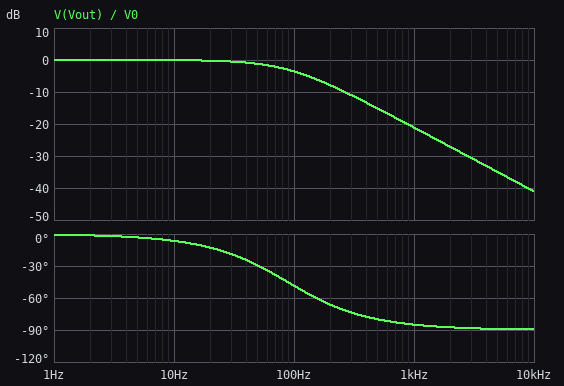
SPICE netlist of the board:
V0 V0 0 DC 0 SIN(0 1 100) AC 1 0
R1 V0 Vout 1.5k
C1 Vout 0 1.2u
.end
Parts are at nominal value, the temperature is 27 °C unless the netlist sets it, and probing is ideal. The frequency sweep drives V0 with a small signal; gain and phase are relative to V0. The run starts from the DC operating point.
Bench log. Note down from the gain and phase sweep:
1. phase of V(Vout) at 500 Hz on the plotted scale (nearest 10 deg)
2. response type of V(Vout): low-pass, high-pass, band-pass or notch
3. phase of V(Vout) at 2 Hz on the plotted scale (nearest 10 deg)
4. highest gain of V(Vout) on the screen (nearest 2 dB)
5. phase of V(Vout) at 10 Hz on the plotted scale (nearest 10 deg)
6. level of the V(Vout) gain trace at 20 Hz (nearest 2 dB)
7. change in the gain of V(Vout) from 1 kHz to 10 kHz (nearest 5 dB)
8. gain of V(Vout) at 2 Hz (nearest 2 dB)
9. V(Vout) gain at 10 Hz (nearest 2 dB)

-80 deg
low-pass
0 deg
0 dB
-10 deg
0 dB
-20 dB
0 dB
0 dB
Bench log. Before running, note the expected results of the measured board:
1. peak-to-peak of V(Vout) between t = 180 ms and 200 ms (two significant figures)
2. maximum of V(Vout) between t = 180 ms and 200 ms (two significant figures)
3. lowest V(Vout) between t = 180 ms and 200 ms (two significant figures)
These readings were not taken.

1.3 V
660 mV
-660 mV
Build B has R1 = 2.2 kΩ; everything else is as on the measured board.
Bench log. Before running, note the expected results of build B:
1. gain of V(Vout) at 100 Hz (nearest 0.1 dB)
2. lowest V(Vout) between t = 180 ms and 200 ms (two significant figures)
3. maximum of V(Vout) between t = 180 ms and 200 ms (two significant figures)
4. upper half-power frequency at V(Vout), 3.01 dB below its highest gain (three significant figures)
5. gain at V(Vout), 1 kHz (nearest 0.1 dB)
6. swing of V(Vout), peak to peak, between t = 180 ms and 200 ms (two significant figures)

-5.7 dB
-520 mV
520 mV
60.3 Hz
-24.4 dB
1.0 V
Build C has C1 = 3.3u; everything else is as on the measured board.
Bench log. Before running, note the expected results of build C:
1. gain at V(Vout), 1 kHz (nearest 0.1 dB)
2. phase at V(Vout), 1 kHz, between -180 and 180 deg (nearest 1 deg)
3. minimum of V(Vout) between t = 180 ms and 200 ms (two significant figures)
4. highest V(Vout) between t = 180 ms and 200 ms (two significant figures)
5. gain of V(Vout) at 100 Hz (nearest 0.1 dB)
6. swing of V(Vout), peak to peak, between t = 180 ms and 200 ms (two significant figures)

-29.9 dB
-88 deg
-310 mV
310 mV
-10.3 dB
610 mV
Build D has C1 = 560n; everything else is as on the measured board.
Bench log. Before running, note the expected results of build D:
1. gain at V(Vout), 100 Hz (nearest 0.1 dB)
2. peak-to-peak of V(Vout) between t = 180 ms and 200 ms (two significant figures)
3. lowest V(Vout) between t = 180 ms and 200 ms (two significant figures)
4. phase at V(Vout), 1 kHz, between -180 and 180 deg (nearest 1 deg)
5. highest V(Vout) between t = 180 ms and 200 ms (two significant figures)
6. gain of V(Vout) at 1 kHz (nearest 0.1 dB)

-1.1 dB
1.8 V
-880 mV
-79 deg
880 mV
-14.6 dB
